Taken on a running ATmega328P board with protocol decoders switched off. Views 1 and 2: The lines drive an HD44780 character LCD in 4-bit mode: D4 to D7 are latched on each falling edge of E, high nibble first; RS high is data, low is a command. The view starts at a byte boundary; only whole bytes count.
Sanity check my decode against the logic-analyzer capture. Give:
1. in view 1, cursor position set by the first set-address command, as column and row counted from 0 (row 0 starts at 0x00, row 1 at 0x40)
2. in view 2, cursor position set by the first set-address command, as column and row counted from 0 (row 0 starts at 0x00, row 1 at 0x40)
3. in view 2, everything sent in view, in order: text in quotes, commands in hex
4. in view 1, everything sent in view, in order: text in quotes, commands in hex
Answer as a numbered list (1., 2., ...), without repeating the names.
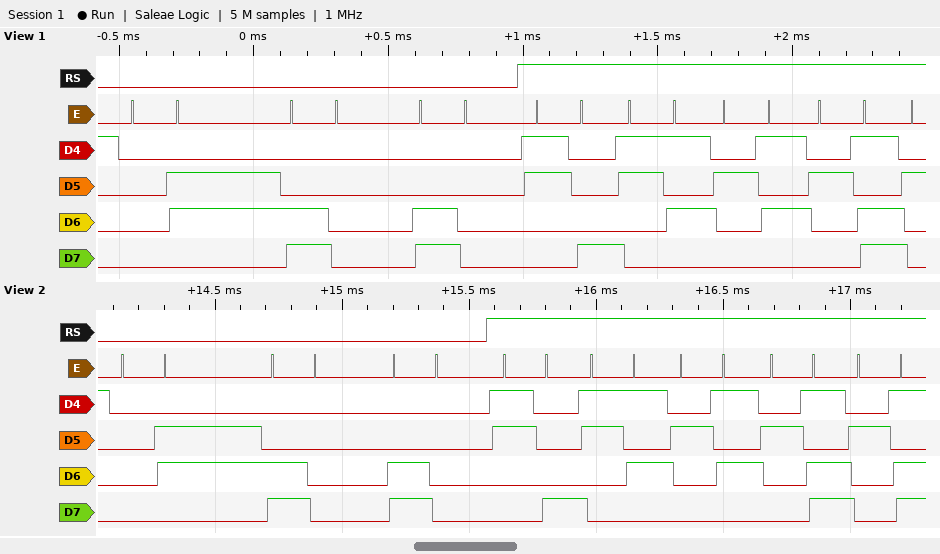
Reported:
1. column 0, row 1
2. column 0, row 1
3. 0x06 0xC0 0xC0 "85%--"
4. 0x06 0xC0 0xC0 "85%-"
